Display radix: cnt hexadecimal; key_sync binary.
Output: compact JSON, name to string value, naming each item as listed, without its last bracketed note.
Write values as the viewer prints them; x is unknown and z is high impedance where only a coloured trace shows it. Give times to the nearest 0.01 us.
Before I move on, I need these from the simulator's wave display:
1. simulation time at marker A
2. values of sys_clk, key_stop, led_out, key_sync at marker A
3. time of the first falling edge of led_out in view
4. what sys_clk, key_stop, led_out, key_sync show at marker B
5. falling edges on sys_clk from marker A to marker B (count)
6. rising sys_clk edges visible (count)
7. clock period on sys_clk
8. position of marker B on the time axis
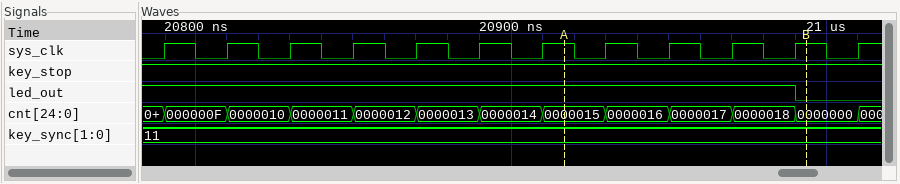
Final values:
{"simulation time at marker A": "20.92 us", "values of sys_clk, key_stop, led_out, key_sync at marker A": "sys_clk=1, key_stop=1, led_out=1, key_sync=11", "time of the first falling edge of led_out in view": "20.99 us", "what sys_clk, key_stop, led_out, key_sync show at marker B": "sys_clk=1, key_stop=1, led_out=0, key_sync=11", "falling edges on sys_clk from marker A to marker B": "4", "rising sys_clk edges visible": "12", "clock period on sys_clk": "0.02 us", "position of marker B on the time axis": "20.99 us"}
